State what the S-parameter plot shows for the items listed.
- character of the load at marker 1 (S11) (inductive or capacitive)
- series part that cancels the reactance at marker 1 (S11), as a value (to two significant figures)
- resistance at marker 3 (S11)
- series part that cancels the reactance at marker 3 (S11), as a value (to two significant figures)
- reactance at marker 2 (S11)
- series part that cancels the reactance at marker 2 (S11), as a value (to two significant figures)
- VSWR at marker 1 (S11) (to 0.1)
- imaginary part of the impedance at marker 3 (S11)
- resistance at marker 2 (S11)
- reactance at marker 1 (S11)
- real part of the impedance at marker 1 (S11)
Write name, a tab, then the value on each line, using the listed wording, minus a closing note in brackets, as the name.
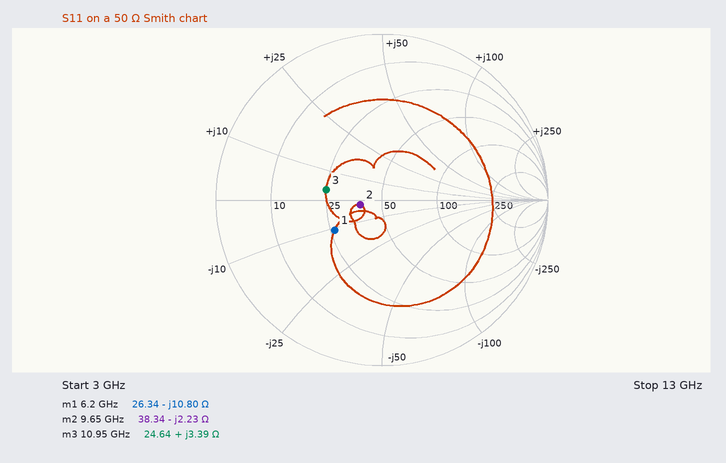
character of the load at marker 1 (S11)	capacitive
series part that cancels the reactance at marker 1 (S11), as a value	280 pH
resistance at marker 3	24.64 Ω
series part that cancels the reactance at marker 3 (S11), as a value	4.3 pF
reactance at marker 2	-2.23 Ω
series part that cancels the reactance at marker 2 (S11), as a value	37 pH
VSWR at marker 1 (S11)	2.0
imaginary part of the impedance at marker 3	+3.39 Ω
resistance at marker 2	38.34 Ω
reactance at marker 1	-10.80 Ω
real part of the impedance at marker 1	26.34 Ω
